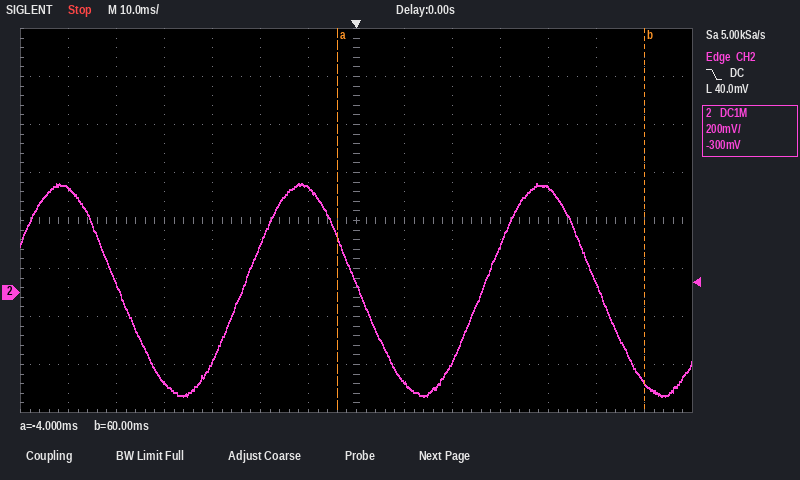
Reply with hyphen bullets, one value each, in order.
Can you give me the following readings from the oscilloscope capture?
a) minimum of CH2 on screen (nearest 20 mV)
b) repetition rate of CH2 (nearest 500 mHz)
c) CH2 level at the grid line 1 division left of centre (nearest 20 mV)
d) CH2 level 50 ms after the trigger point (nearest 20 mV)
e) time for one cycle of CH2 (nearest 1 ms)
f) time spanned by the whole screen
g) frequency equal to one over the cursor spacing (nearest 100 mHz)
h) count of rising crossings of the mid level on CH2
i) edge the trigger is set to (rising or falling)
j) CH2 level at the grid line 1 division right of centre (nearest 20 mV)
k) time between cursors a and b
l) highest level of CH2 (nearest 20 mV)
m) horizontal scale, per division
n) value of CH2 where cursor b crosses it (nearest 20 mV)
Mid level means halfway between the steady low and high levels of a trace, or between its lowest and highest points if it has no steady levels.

- -440 mV
- 20.0 Hz
- 440 mV
- 40 mV
- 50 ms
- 140 ms
- 15.6 Hz
- 2
- falling
- -380 mV
- 64 ms
- 460 mV
- 10 ms
- -380 mV
